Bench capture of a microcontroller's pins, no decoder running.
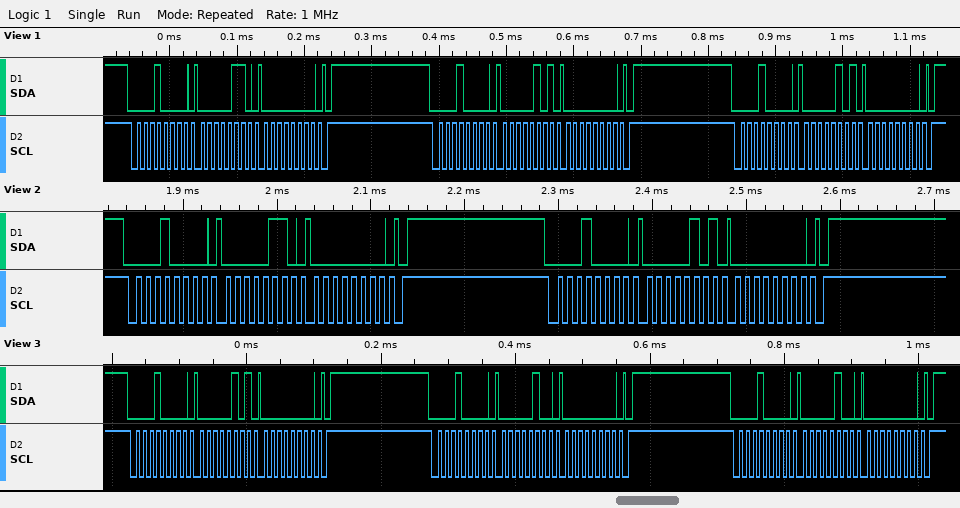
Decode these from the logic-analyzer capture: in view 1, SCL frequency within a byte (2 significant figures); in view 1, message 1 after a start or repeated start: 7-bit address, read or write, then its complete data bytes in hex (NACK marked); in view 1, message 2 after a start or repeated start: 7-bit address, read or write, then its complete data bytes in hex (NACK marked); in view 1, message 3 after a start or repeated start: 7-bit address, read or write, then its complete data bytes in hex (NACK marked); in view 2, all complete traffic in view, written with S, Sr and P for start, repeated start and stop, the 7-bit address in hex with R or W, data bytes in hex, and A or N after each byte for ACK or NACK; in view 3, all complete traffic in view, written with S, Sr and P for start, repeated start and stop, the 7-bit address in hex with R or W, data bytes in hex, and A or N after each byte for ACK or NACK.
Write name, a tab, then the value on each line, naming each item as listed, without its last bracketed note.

in view 1, SCL frequency within a byte	100 kHz
in view 1, message 1 after a start or repeated start: 7-bit address, read or write, then its complete data bytes in hex	0x08 write: 06 00
in view 1, message 2 after a start or repeated start: 7-bit address, read or write, then its complete data bytes in hex	0x08 write: 05 00
in view 1, message 3 after a start or repeated start: 7-bit address, read or write, then its complete data bytes in hex	0x08 write: 05 00
in view 2, all complete traffic in view, written with S, Sr and P for start, repeated start and stop, the 7-bit address in hex with R or W, data bytes in hex, and A or N after each byte for ACK or NACK	S 08W A 06 A 00 A P S 08W A 05 A 00 A P
in view 3, all complete traffic in view, written with S, Sr and P for start, repeated start and stop, the 7-bit address in hex with R or W, data bytes in hex, and A or N after each byte for ACK or NACK	S 08W A 05 A 00 A P S 08W A 04 A 00 A P S 08W A 04 A 00 A P
